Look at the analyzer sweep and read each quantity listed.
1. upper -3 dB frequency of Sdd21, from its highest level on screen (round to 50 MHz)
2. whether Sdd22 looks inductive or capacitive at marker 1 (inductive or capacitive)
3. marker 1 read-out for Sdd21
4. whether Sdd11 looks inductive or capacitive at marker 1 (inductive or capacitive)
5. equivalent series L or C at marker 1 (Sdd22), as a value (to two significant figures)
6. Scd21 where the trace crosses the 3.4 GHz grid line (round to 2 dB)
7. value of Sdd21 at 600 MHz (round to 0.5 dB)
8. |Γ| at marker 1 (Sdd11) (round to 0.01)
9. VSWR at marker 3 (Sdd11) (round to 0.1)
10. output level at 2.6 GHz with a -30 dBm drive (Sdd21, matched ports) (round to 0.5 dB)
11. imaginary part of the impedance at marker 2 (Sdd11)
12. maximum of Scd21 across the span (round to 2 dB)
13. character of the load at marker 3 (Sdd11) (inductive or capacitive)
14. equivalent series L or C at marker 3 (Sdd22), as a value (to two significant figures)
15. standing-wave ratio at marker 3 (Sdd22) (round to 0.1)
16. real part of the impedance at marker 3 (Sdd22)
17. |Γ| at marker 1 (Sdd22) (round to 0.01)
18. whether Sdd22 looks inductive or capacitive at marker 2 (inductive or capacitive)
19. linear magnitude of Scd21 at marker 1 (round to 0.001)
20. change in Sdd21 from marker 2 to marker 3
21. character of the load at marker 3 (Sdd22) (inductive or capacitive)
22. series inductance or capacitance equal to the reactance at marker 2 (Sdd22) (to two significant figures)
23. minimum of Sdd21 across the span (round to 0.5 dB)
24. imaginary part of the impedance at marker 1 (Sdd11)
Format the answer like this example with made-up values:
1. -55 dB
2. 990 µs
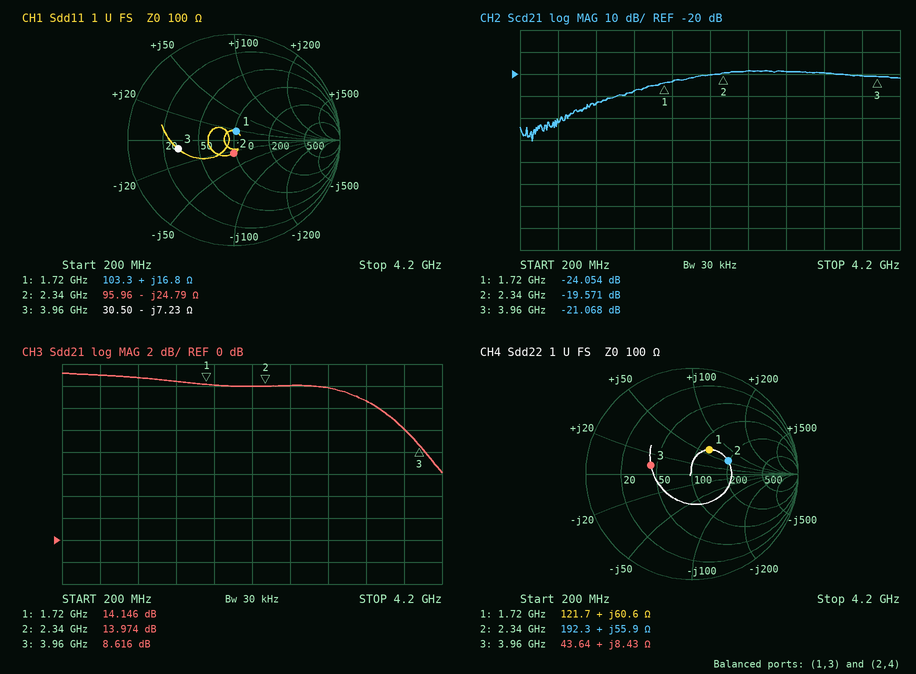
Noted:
1. 3.50 GHz
2. inductive
3. 14.146 dB
4. inductive
5. 5.6 nH
6. -20 dB
7. 15.0 dB
8. 0.08
9. 3.3
10. -16.0 dBm
11. -24.79 Ω
12. -18 dB
13. capacitive
14. 340 pH
15. 2.3
16. 43.64 Ω
17. 0.28
18. inductive
19. 0.063
20. -5.358 dB
21. inductive
22. 3.8 nH
23. 6.0 dB
24. +16.8 Ω
